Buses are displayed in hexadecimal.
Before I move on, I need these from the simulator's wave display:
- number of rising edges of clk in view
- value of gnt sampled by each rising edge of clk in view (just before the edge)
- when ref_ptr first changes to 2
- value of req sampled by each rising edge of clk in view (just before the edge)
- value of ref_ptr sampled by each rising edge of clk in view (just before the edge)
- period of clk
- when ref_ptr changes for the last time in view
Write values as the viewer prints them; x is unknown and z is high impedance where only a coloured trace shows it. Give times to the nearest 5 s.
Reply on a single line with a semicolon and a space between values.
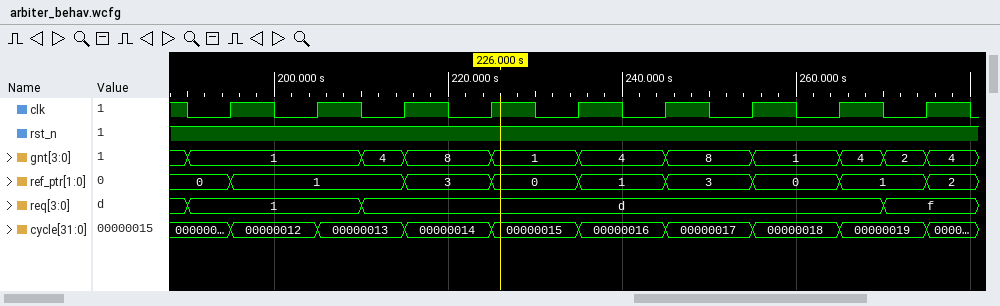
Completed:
9; 1, 1, 4, 8, 1, 4, 8, 1, 2; 275 s; 1, 1, d, d, d, d, d, d, f; 0, 1, 1, 3, 0, 1, 3, 0, 1; 10 s; 275 s
